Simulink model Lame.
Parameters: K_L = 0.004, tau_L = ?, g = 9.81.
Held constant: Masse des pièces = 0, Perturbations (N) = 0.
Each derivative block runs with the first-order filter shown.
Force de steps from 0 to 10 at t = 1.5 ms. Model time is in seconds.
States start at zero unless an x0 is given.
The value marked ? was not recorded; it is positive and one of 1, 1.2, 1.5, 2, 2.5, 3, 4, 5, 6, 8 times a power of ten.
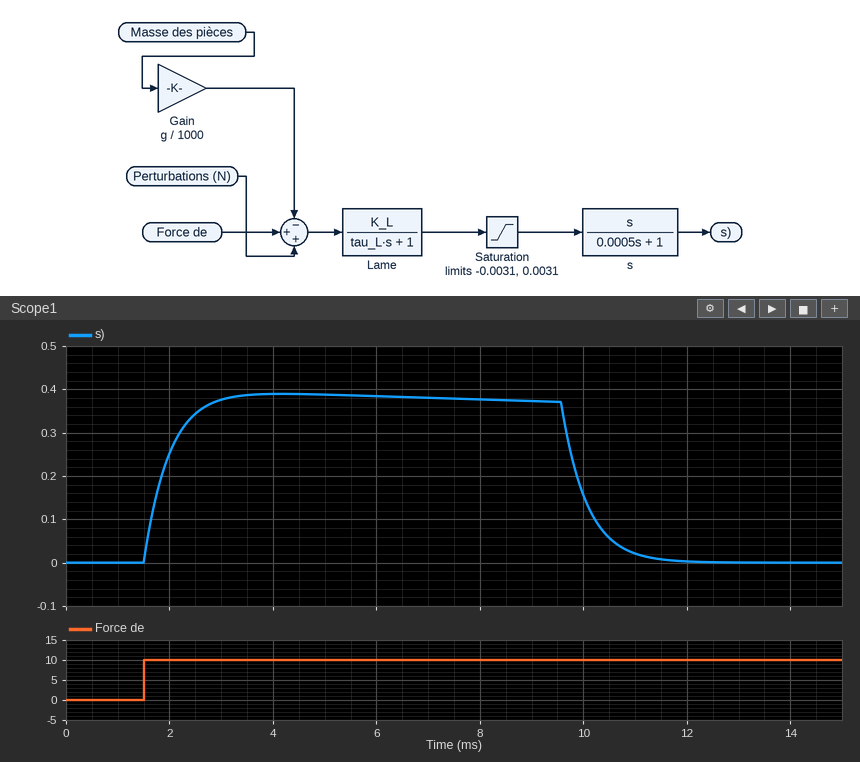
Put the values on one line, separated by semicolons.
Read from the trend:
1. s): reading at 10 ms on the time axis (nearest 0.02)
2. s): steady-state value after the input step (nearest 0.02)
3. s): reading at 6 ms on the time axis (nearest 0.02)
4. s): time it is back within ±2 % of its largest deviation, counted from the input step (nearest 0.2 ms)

0.16; 0.00; 0.38; 10.0 ms
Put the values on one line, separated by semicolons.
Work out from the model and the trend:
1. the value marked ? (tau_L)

0.1
